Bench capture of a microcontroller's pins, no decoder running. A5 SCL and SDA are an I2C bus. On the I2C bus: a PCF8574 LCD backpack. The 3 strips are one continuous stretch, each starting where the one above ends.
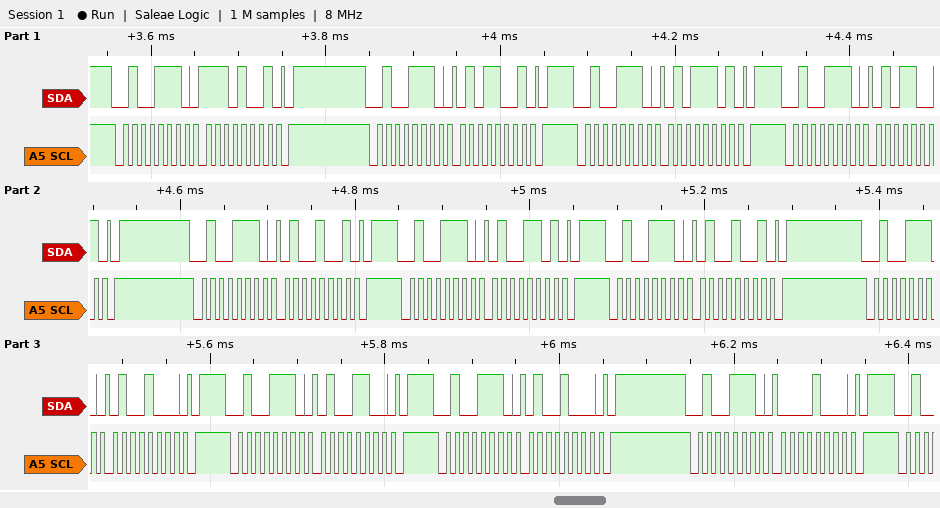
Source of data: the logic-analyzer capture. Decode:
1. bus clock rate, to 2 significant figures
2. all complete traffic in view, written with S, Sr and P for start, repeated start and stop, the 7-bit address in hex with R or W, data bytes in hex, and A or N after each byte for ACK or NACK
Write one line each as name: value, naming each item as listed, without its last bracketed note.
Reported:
bus clock rate, to 2 significant figures: 100 kHz
all complete traffic in view, written with S, Sr and P for start, repeated start and stop, the 7-bit address in hex with R or W, data bytes in hex, and A or N after each byte for ACK or NACK: S 27W A E9 A P S 27W A 59 A P S 27W A 5D A P S 27W A 59 A P S 27W A 49 A P S 27W A 4D A P S 27W A 49 A P S 27W A 48 A P S 27W A 4C A P S 27W A 48 A P S 27W A 08 A P
